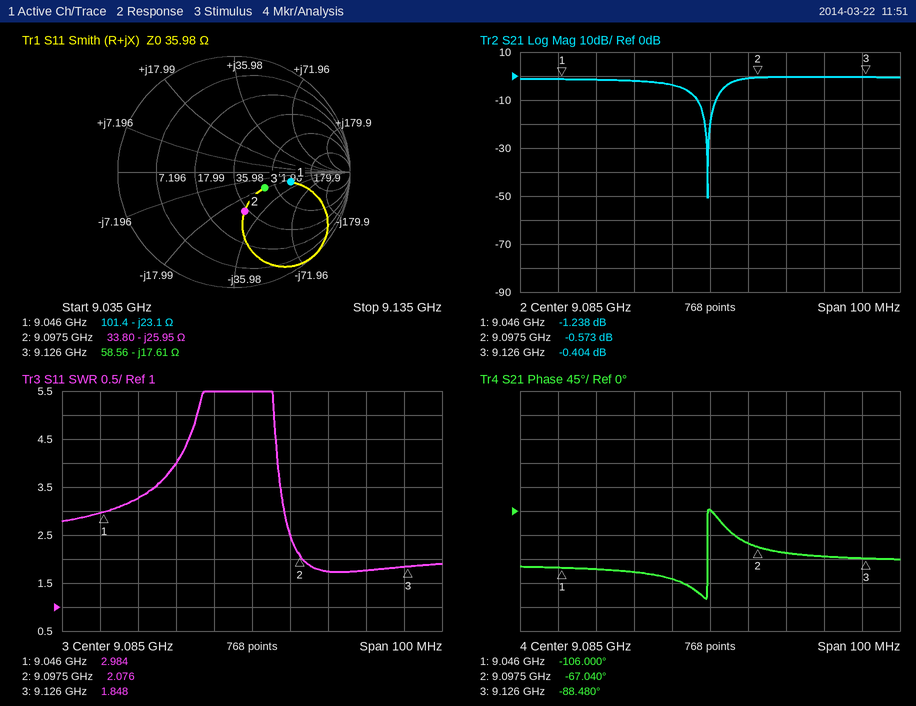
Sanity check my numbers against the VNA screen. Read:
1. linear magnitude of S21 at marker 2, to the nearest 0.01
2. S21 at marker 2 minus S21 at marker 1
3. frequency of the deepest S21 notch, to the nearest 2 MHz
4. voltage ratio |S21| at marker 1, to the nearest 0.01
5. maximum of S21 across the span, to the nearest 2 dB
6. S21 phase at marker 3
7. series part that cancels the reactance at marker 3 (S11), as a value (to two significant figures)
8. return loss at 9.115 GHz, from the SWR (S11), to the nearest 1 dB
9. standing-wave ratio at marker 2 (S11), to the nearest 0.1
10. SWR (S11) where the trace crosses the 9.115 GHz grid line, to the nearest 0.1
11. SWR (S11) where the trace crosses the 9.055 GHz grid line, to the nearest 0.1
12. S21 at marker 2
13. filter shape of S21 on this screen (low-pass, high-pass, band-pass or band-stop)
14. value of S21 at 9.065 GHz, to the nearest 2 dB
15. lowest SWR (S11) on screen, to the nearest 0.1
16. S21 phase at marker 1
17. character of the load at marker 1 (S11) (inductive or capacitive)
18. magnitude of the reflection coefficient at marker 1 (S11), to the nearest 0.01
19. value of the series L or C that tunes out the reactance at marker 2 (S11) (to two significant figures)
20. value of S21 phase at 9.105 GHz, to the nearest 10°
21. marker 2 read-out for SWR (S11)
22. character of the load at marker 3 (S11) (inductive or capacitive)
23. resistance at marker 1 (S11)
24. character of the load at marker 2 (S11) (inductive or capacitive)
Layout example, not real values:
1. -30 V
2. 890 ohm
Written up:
1. 0.94
2. 0.665 dB
3. 9.084 GHz
4. 0.87
5. 0 dB
6. -88.480°
7. 310 pH
8. 11 dB
9. 2.1
10. 1.8
11. 3.3
12. -0.573 dB
13. band-stop
14. -2 dB
15. 1.7
16. -106.000°
17. capacitive
18. 0.50
19. 450 pH
20. -80°
21. 2.076
22. capacitive
23. 101.4 Ω
24. capacitive
